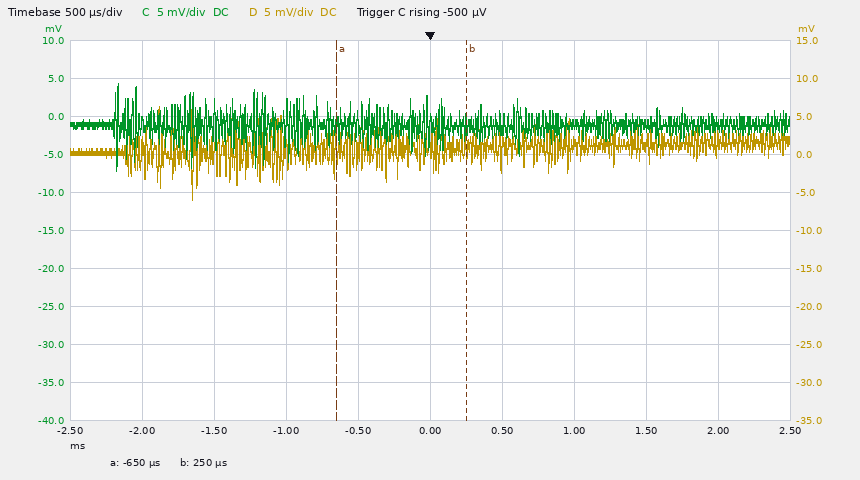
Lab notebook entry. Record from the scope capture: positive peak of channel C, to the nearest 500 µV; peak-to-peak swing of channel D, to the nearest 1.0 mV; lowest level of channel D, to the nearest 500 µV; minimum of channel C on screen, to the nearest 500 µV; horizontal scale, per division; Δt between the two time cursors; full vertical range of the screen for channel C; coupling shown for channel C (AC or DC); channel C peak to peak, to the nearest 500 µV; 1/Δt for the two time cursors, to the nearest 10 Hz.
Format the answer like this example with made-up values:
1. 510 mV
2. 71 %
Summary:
1. 4.5 mV
2. 12.0 mV
3. -6.0 mV
4. -7.0 mV
5. 500 µs
6. 900 µs
7. 50 mV
8. DC
9. 11.5 mV
10. 1.11 kHz
